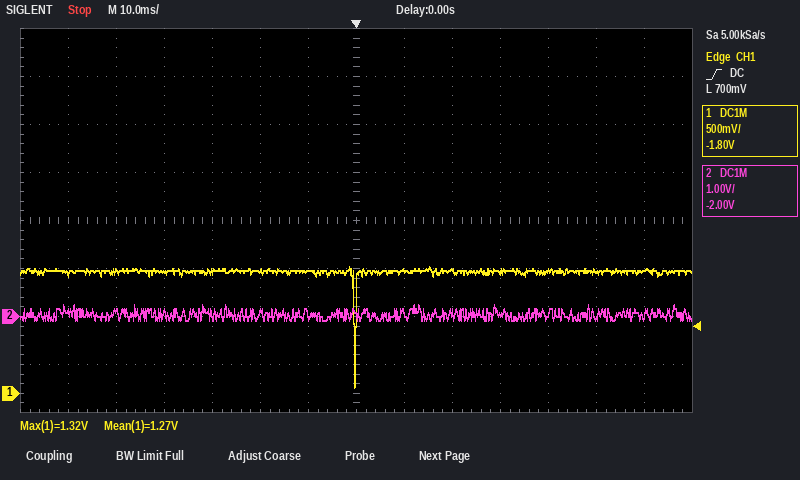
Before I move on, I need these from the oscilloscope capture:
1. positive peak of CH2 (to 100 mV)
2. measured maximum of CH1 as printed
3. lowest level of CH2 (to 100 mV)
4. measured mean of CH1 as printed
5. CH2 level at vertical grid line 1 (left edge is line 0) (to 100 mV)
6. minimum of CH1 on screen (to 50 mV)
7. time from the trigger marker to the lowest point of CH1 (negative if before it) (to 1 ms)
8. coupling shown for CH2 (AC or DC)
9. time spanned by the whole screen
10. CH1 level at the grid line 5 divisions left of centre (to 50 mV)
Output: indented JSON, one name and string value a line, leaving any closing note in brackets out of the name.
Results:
{
  "positive peak of CH2": "200 mV",
  "measured maximum of CH1 as printed": "1.32 V",
  "lowest level of CH2": "-100 mV",
  "measured mean of CH1 as printed": "1.27 V",
  "CH2 level at vertical grid line 1 (left edge is line 0)": "100 mV",
  "minimum of CH1 on screen": "50 mV",
  "time from the trigger marker to the lowest point of CH1 (negative if before it)": "0 ms",
  "coupling shown for CH2": "DC",
  "time spanned by the whole screen": "140 ms",
  "CH1 level at the grid line 5 divisions left of centre": "1.25 V"
}
